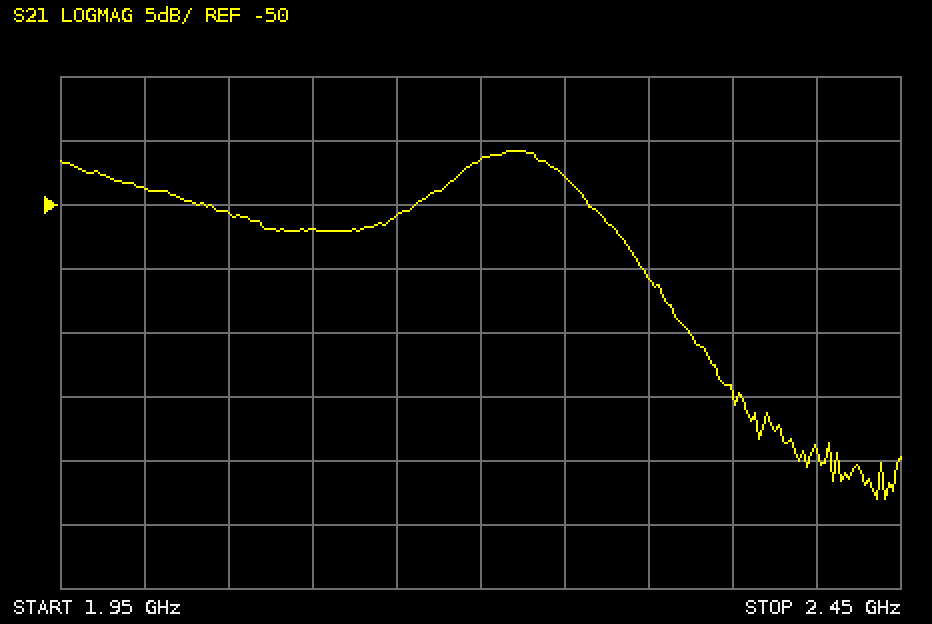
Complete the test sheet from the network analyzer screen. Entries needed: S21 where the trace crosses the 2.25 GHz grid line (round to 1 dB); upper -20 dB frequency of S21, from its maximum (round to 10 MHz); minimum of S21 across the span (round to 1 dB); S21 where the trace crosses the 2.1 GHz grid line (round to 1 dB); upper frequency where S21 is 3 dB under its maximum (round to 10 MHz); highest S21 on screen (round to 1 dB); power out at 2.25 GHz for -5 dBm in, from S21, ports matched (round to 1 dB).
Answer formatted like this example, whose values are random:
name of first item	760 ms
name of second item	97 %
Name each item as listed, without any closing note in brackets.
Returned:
S21 where the trace crosses the 2.25 GHz grid line	-48 dB
upper -20 dB frequency of S21, from its maximum	2.36 GHz
minimum of S21 across the span	-73 dB
S21 where the trace crosses the 2.1 GHz grid line	-52 dB
upper frequency where S21 is 3 dB under its maximum	2.26 GHz
highest S21 on screen	-46 dB
power out at 2.25 GHz for -5 dBm in, from S21, ports matched	-53 dBm
